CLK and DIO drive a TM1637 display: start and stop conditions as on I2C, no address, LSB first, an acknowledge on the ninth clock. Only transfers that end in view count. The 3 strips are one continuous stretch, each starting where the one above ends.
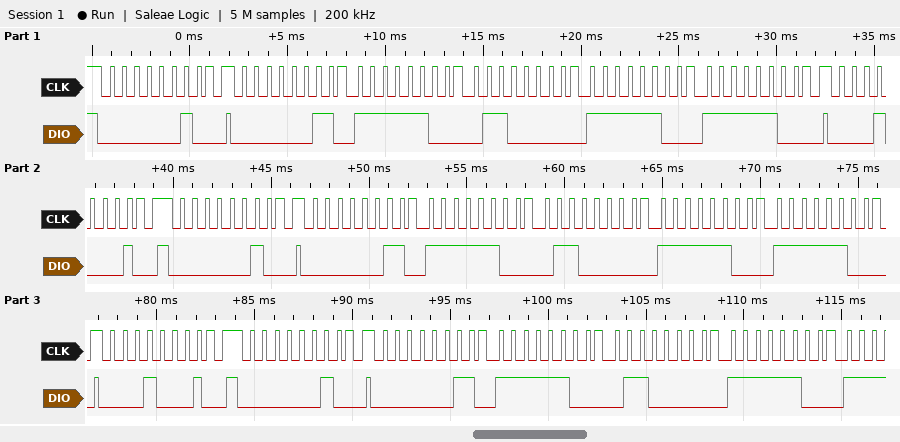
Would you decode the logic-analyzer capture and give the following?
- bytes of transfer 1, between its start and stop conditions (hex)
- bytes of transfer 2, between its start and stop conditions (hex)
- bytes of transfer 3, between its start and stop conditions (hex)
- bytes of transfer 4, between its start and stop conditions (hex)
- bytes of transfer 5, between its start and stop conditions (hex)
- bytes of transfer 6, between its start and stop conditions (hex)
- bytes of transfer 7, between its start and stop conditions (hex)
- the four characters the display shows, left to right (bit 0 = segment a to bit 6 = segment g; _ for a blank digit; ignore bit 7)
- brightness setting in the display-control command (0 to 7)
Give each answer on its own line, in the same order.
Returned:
40
C0 3F 06 3F 3F
88
40
C0 3F 06 3F 3F
88
40
0100
0
